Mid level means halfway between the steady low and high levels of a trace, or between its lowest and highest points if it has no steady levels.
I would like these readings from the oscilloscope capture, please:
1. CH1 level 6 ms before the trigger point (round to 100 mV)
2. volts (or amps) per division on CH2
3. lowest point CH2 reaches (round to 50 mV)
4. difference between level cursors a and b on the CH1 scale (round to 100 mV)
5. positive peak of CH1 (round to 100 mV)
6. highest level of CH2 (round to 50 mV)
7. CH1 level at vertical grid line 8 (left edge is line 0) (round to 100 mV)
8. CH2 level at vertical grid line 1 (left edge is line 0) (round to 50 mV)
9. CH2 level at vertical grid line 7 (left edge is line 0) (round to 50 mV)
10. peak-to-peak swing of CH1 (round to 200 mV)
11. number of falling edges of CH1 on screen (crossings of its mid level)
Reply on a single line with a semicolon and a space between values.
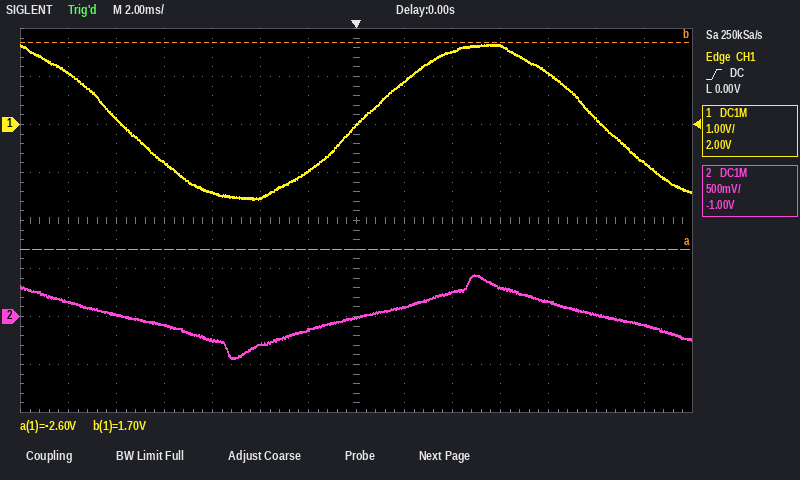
-1.4 V; 500 mV; -450 mV; 4.3 V; 1.7 V; 450 mV; 900 mV; 150 mV; 0 mV; 3.2 V; 2
